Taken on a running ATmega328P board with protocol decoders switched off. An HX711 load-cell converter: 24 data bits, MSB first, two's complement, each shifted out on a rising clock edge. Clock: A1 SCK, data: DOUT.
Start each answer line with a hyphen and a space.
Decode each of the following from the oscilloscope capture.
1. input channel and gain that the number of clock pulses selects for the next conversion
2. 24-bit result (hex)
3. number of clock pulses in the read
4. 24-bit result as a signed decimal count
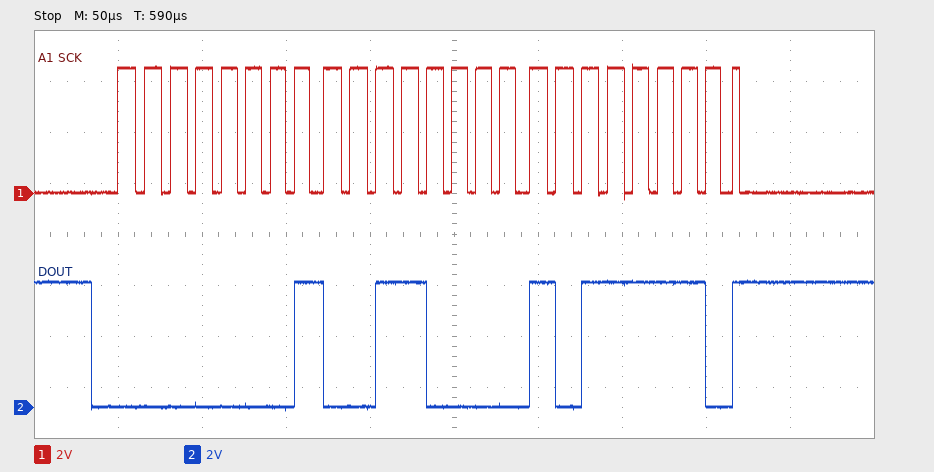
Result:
- channel A, gain 128
- 0x0130BE
- 25
- 78014
